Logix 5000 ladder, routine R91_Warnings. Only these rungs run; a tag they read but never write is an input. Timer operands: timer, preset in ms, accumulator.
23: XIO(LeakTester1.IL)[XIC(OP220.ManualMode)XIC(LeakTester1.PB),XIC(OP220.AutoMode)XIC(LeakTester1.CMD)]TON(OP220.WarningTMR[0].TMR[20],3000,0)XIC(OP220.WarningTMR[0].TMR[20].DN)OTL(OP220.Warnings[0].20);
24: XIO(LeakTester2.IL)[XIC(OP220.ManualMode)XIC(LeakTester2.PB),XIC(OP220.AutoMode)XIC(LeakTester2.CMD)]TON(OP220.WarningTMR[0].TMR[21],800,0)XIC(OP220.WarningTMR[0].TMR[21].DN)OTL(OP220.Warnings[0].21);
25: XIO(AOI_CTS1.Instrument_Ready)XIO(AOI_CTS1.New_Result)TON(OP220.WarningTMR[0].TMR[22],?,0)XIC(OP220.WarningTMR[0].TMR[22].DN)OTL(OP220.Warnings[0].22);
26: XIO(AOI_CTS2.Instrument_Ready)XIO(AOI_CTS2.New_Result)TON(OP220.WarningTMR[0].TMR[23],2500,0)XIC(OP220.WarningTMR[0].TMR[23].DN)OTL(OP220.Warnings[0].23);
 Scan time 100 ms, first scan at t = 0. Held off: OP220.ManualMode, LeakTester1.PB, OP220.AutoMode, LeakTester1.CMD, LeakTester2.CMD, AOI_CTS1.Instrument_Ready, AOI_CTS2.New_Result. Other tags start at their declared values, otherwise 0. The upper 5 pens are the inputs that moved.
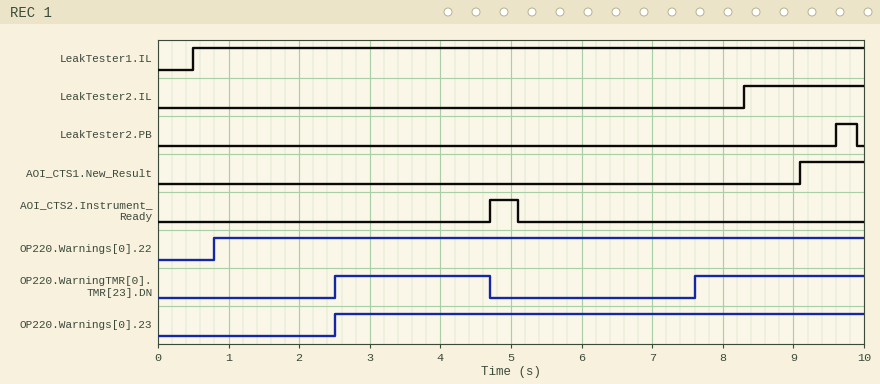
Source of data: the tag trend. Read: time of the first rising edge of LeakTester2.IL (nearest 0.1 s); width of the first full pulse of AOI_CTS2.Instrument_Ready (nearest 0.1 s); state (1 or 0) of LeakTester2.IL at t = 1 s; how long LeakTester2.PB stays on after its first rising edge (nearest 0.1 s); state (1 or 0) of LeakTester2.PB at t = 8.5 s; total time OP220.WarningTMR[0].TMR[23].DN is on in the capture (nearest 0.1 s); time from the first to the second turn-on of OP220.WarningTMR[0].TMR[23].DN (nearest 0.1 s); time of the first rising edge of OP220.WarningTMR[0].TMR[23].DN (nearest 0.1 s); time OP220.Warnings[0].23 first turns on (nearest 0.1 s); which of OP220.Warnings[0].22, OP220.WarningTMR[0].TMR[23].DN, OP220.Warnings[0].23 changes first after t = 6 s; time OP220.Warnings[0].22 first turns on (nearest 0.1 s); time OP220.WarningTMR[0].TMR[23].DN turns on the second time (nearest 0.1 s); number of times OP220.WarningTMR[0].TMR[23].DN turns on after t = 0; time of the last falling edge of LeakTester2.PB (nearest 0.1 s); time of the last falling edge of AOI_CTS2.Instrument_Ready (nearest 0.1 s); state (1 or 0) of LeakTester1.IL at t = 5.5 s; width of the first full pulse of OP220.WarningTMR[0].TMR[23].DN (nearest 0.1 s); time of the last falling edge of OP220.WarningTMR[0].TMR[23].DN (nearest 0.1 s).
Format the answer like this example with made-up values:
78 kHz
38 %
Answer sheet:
8.3 s
0.4 s
0
0.3 s
0
4.6 s
5.1 s
2.5 s
2.5 s
OP220.WarningTMR[0].TMR[23].DN
0.8 s
7.6 s
2
9.9 s
5.1 s
1
2.2 s
4.7 s
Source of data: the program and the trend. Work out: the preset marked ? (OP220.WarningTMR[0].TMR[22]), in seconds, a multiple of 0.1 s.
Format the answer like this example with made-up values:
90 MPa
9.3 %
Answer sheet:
0.8 s
